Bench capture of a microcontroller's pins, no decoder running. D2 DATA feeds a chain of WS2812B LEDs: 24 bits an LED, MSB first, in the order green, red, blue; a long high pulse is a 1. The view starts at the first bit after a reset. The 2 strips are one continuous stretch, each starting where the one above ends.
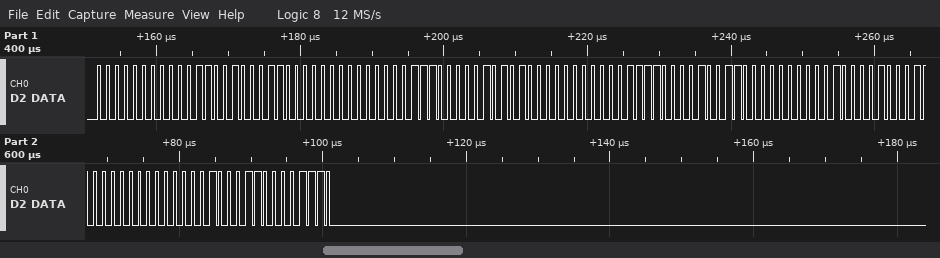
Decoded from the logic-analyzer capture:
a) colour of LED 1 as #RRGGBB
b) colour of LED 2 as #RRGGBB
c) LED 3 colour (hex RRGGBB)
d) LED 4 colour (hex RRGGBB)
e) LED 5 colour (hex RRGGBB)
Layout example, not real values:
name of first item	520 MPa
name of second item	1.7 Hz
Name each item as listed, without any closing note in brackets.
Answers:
colour of LED 1 as #RRGGBB	#190018
colour of LED 2 as #RRGGBB	#1C0015
LED 3 colour	#1E0013
LED 4 colour	#210010
LED 5 colour	#23000E
